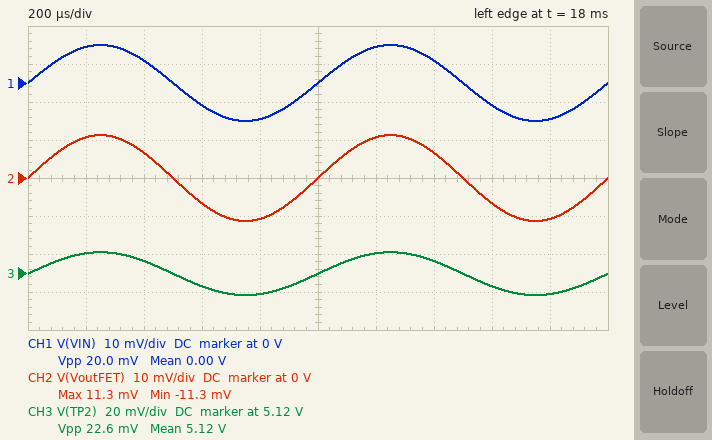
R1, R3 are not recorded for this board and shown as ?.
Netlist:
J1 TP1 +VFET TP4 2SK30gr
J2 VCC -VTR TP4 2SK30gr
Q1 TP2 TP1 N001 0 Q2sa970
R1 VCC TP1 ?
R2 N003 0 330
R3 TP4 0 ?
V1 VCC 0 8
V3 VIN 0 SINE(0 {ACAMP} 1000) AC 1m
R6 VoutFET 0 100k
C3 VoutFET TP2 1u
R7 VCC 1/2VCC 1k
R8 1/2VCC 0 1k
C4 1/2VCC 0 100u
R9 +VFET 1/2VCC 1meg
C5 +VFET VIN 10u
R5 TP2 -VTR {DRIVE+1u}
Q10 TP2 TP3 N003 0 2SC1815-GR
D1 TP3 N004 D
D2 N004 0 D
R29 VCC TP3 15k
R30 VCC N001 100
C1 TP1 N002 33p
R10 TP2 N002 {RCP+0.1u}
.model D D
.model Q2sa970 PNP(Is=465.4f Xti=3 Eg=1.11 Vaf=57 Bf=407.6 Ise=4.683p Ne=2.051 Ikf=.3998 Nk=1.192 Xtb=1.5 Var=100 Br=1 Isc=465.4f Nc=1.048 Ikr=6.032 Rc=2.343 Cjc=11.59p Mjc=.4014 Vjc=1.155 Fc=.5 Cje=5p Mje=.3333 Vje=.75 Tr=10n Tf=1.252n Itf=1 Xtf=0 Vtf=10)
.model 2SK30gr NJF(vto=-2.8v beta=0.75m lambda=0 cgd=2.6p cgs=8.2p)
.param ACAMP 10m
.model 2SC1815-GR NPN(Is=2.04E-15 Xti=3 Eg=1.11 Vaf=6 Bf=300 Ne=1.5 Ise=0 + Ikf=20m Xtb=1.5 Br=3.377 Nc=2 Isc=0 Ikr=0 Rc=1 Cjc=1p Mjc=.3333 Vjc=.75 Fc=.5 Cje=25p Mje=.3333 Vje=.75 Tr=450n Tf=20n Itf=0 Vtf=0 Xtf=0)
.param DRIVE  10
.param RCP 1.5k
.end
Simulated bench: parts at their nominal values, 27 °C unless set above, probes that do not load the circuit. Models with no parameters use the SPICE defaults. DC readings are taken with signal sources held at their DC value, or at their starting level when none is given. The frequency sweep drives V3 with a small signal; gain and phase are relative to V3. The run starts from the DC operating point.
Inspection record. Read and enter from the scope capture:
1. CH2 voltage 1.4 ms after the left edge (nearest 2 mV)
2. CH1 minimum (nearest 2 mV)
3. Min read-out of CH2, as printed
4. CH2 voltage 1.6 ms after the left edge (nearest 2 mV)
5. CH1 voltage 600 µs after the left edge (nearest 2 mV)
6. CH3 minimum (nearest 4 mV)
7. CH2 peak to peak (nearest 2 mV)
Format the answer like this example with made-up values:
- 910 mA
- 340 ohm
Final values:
- 6 mV
- -10 mV
- -11.3 mV
- -6 mV
- -6 mV
- 5.108 V
- 22 mV
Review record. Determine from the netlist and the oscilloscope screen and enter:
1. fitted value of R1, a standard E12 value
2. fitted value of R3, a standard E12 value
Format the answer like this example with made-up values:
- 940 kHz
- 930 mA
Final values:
- 5.6 kΩ
- 3.3 kΩ
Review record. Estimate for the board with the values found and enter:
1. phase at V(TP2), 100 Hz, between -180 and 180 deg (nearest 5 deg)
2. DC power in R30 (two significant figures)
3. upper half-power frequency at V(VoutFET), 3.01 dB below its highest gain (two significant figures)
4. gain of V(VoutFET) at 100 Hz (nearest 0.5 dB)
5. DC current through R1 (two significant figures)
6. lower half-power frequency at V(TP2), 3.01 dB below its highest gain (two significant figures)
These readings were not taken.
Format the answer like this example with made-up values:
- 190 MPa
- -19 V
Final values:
- 0 deg
- 300 µW
- 1.4 MHz
- 1.0 dB
- 130 µA
- 16 mHz
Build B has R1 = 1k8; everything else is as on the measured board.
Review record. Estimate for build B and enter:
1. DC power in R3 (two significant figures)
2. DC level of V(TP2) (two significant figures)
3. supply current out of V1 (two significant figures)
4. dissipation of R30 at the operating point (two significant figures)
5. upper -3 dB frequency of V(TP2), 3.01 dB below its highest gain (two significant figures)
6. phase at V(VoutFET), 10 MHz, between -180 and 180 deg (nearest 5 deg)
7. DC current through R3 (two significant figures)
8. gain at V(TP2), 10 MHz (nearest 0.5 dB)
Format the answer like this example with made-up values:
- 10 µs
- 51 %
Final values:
- 11 mW
- 4.6 V
- 8.0 mA
- 300 µW
- 2.0 MHz
- -45 deg
- 1.8 mA
- -6.0 dB
